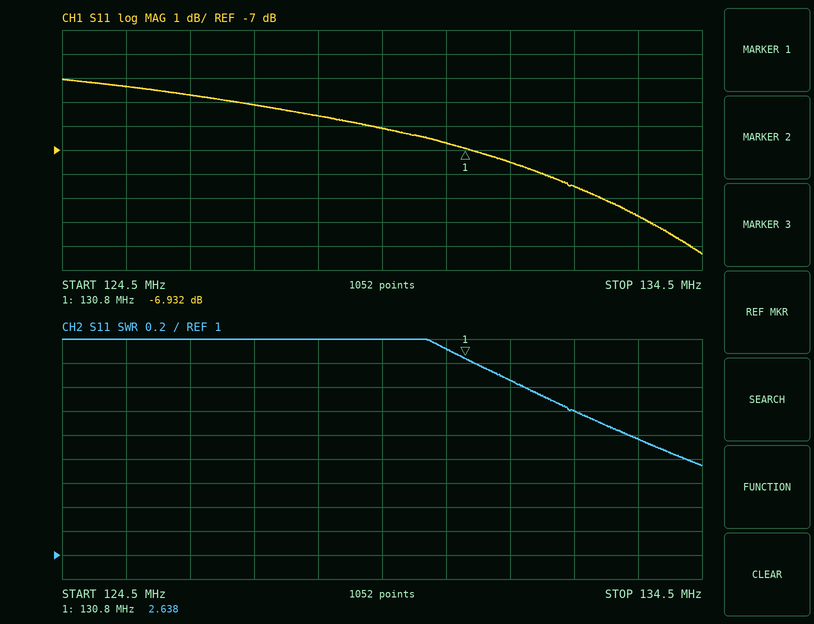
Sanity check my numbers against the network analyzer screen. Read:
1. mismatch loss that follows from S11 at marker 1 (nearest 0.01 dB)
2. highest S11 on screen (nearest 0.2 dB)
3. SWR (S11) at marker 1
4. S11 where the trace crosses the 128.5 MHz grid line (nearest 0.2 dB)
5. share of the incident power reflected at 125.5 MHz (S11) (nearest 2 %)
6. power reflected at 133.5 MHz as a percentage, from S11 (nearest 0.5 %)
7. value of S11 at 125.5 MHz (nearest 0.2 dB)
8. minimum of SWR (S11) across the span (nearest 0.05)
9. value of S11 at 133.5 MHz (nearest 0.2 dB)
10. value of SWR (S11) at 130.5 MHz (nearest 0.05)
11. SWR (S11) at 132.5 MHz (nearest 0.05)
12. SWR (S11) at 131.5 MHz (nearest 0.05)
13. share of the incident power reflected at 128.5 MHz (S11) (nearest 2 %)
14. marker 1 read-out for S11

0.98 dB
-4.0 dB
2.638
-5.6 dB
36 %
10.5 %
-4.4 dB
1.75
-9.8 dB
2.70
2.20
2.45
28 %
-6.932 dB
